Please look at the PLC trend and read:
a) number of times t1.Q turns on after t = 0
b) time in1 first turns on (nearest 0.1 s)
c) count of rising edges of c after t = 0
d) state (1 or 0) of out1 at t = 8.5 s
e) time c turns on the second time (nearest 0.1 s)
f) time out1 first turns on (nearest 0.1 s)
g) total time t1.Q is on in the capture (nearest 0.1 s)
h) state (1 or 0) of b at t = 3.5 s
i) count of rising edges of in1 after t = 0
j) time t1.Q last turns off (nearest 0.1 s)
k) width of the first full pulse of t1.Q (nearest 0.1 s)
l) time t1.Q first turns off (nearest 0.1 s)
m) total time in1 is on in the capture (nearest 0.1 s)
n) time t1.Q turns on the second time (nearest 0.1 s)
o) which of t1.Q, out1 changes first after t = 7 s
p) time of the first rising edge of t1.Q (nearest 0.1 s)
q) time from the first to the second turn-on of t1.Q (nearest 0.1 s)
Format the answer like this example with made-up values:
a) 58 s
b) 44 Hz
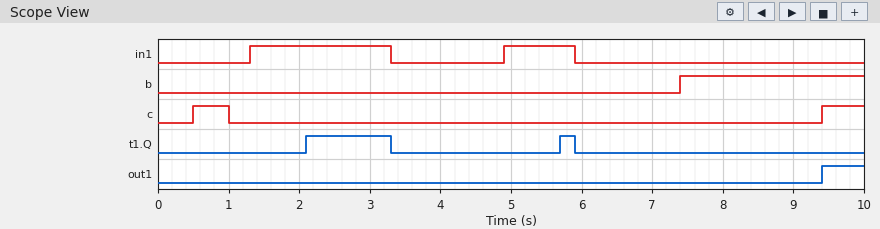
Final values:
a) 2
b) 1.3 s
c) 2
d) 0
e) 9.4 s
f) 9.4 s
g) 1.4 s
h) 0
i) 2
j) 5.9 s
k) 1.2 s
l) 3.3 s
m) 3.0 s
n) 5.7 s
o) out1
p) 2.1 s
q) 3.6 s
